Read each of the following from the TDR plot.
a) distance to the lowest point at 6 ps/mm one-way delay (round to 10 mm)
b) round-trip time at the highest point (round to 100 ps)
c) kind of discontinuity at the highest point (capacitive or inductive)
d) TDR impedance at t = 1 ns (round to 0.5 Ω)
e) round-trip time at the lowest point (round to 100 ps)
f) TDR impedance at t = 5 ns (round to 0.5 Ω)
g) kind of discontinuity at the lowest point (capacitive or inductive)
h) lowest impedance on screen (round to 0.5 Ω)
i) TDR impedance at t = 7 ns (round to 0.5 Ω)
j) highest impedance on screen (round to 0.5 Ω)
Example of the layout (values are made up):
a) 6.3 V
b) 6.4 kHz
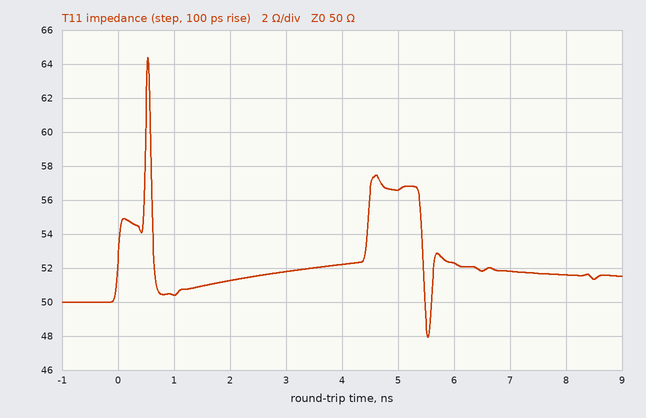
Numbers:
a) 460 mm
b) 500 ps
c) inductive
d) 50.5 Ω
e) 5.5 ns
f) 56.5 Ω
g) capacitive
h) 48.0 Ω
i) 52.0 Ω
j) 64.5 Ω
